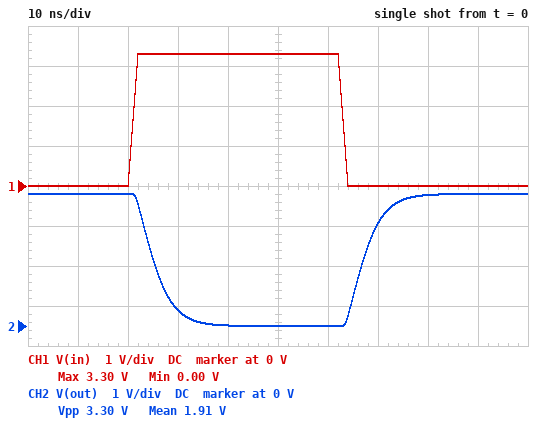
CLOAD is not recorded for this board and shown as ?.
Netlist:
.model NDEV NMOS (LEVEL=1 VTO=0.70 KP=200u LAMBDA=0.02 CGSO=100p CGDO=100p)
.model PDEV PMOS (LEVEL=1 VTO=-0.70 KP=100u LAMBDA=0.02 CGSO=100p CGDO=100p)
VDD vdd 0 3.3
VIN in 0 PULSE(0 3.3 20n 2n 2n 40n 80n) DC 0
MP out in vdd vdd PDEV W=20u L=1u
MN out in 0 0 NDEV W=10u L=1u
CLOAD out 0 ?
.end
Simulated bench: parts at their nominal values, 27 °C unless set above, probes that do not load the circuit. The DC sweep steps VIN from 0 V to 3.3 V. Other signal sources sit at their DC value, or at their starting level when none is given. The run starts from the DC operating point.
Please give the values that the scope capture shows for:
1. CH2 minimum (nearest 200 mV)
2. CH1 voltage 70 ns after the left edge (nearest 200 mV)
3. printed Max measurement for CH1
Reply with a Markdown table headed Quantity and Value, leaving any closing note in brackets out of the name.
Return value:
| Quantity | Value |
|---|---|
| CH2 minimum | 0 V |
| CH1 voltage 70 ns after the left edge | 0 V |
| printed Max measurement for CH1 | 3.30 V |
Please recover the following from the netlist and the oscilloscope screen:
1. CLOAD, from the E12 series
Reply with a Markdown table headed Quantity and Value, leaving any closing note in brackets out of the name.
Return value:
| Quantity | Value |
|---|---|
| CLOAD, from the E12 series | 15 pF |
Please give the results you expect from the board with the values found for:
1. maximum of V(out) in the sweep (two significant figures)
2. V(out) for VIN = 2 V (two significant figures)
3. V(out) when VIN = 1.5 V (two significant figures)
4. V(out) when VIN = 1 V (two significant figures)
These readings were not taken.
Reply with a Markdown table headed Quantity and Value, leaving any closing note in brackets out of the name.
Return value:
| Quantity | Value |
|---|---|
| maximum of V(out) in the sweep | 3.3 V |
| V(out) for VIN = 2 V | 160 mV |
| V(out) when VIN = 1.5 V | 2.9 V |
| V(out) when VIN = 1 V | 3.3 V |
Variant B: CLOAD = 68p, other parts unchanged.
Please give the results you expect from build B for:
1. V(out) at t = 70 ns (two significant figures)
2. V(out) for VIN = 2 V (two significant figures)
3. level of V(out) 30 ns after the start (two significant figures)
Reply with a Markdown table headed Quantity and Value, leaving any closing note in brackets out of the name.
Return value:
| Quantity | Value |
|---|---|
| V(out) at t = 70 ns | 1.0 V |
| V(out) for VIN = 2 V | 160 mV |
| level of V(out) 30 ns after the start | 2.4 V |
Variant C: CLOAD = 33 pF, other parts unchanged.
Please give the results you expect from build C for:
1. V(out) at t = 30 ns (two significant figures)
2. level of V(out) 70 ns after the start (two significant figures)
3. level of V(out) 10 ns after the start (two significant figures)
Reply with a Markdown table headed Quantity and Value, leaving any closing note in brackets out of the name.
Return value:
| Quantity | Value |
|---|---|
| V(out) at t = 30 ns | 1.5 V |
| level of V(out) 70 ns after the start | 1.4 V |
| level of V(out) 10 ns after the start | 3.3 V |
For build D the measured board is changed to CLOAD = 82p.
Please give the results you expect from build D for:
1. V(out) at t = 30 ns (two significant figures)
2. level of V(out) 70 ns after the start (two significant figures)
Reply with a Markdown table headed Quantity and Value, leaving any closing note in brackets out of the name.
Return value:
| Quantity | Value |
|---|---|
| V(out) at t = 30 ns | 2.6 V |
| level of V(out) 70 ns after the start | 1.1 V |
